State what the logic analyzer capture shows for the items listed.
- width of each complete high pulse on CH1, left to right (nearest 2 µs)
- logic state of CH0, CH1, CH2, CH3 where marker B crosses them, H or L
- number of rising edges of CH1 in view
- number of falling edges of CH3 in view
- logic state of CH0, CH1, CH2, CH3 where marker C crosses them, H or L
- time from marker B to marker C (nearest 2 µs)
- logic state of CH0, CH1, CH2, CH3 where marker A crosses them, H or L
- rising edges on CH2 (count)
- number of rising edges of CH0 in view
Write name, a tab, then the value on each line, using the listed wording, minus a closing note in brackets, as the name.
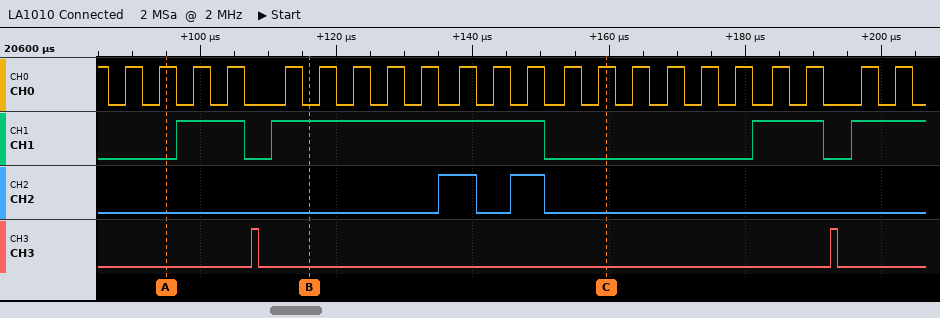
width of each complete high pulse on CH1, left to right	10 µs, 40 µs, 10 µs
logic state of CH0, CH1, CH2, CH3 where marker B crosses them, H or L	CH0=L, CH1=H, CH2=L, CH3=L
number of rising edges of CH1 in view	4
number of falling edges of CH3 in view	2
logic state of CH0, CH1, CH2, CH3 where marker C crosses them, H or L	CH0=H, CH1=L, CH2=L, CH3=L
time from marker B to marker C	44 µs
logic state of CH0, CH1, CH2, CH3 where marker A crosses them, H or L	CH0=H, CH1=L, CH2=L, CH3=L
rising edges on CH2	2
number of rising edges of CH0 in view	22
